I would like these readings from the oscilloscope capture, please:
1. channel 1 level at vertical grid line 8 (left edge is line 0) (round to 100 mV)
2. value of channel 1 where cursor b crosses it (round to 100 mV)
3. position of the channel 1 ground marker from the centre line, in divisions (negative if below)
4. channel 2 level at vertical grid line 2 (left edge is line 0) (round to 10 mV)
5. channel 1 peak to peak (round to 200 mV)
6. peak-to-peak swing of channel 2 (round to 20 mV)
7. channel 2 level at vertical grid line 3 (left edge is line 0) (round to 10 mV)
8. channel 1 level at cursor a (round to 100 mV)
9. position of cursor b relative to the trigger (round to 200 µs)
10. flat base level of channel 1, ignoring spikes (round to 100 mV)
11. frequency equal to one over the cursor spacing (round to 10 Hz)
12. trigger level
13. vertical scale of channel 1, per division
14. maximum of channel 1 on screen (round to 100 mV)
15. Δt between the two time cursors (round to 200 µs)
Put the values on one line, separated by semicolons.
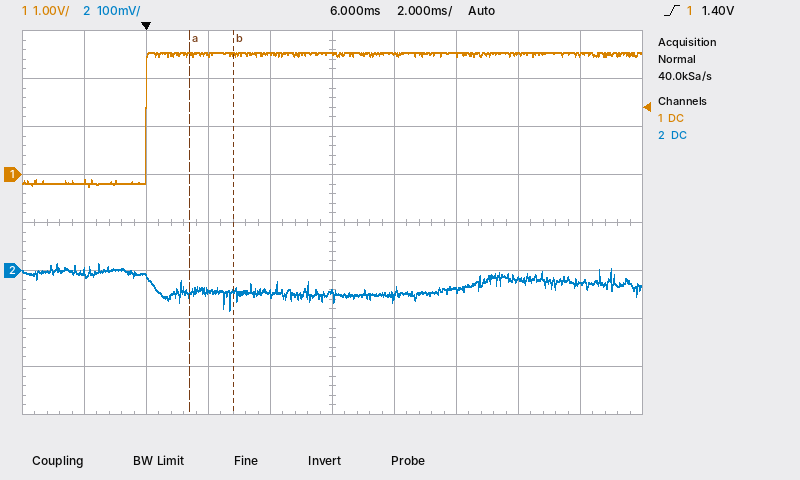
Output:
2.5 V; 2.5 V; +1.0 div; -10 mV; 2.8 V; 100 mV; -40 mV; 2.5 V; +2.8 ms; -200 mV; 710 Hz; 1.40 V; 1 V; 2.5 V; 1.4 ms
